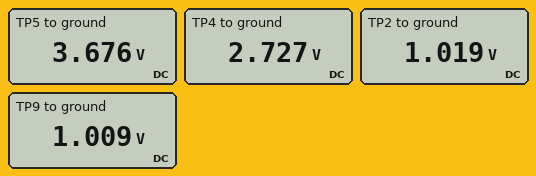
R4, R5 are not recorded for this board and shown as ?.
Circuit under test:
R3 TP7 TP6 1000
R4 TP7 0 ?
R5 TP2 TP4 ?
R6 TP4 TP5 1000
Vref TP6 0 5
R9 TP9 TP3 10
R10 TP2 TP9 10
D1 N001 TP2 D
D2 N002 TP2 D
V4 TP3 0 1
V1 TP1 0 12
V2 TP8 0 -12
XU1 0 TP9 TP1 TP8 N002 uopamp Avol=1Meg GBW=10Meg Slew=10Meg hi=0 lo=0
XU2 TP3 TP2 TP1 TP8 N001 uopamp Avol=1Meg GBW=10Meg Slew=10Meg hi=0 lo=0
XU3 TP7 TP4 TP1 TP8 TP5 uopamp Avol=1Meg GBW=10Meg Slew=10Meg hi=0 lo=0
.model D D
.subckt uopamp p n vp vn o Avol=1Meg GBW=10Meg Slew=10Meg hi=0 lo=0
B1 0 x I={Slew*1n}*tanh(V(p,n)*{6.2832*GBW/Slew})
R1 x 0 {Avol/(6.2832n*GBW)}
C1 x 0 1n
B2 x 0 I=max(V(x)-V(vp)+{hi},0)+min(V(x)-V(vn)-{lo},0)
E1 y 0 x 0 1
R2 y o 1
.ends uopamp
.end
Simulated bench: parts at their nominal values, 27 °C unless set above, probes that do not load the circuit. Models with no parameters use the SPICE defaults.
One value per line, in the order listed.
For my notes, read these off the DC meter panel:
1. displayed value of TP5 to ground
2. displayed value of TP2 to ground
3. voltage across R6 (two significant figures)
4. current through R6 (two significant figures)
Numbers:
3.676 V
1.019 V
950 mV
950 µA
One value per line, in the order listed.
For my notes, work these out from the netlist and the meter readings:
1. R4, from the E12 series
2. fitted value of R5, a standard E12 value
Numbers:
1.2 kΩ
1.8 kΩ
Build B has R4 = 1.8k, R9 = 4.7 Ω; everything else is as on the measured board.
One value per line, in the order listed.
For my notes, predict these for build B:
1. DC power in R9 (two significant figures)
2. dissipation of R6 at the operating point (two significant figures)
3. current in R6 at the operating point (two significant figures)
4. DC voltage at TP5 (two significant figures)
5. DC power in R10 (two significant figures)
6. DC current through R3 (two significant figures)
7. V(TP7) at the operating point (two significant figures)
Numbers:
7.0 µW
1.5 mW
1.2 mA
4.4 V
15 µW
1.8 mA
3.2 V
